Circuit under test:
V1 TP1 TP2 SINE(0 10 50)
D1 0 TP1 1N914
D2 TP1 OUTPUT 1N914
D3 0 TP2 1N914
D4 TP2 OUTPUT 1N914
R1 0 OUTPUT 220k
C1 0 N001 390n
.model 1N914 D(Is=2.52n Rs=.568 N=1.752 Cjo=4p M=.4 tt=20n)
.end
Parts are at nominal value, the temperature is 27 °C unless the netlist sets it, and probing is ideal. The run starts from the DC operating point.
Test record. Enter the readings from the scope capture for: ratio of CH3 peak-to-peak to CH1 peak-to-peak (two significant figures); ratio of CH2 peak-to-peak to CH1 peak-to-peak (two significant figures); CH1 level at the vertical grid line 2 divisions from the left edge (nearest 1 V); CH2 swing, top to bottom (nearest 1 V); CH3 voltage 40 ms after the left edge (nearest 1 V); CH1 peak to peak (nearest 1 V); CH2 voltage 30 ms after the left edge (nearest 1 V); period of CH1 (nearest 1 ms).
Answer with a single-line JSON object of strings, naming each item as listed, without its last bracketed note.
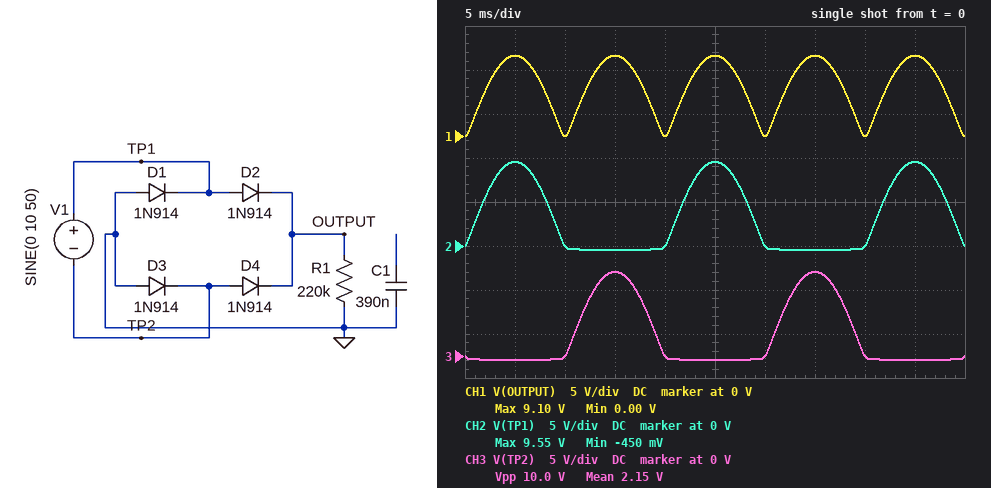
{"ratio of CH3 peak-to-peak to CH1 peak-to-peak": "1.1", "ratio of CH2 peak-to-peak to CH1 peak-to-peak": "1.1", "CH1 level at the vertical grid line 2 divisions from the left edge": "0 V", "CH2 swing, top to bottom": "10 V", "CH3 voltage 40 ms after the left edge": "0 V", "CH1 peak to peak": "9 V", "CH2 voltage 30 ms after the left edge": "0 V", "period of CH1": "10 ms"}
